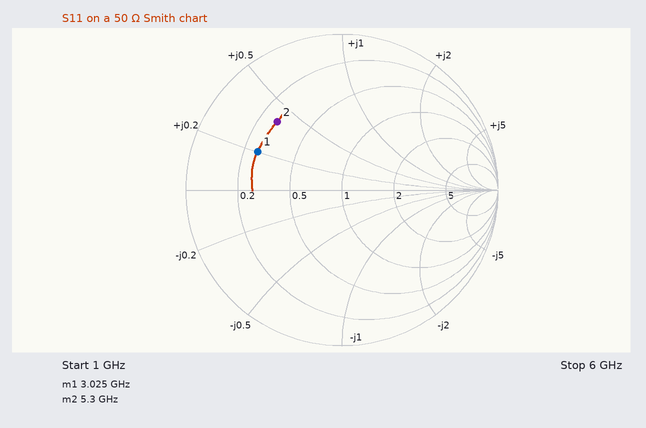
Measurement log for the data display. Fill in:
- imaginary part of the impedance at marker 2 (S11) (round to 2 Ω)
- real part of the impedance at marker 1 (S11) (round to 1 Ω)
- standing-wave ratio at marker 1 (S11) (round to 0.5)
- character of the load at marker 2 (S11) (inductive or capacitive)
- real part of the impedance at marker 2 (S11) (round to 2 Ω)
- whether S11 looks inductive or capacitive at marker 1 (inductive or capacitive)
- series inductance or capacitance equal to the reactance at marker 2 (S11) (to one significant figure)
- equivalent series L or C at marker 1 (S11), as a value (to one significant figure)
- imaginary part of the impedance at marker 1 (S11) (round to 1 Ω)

+20 Ω
13 Ω
4.0
inductive
14 Ω
inductive
600 pH
500 pH
+10 Ω
